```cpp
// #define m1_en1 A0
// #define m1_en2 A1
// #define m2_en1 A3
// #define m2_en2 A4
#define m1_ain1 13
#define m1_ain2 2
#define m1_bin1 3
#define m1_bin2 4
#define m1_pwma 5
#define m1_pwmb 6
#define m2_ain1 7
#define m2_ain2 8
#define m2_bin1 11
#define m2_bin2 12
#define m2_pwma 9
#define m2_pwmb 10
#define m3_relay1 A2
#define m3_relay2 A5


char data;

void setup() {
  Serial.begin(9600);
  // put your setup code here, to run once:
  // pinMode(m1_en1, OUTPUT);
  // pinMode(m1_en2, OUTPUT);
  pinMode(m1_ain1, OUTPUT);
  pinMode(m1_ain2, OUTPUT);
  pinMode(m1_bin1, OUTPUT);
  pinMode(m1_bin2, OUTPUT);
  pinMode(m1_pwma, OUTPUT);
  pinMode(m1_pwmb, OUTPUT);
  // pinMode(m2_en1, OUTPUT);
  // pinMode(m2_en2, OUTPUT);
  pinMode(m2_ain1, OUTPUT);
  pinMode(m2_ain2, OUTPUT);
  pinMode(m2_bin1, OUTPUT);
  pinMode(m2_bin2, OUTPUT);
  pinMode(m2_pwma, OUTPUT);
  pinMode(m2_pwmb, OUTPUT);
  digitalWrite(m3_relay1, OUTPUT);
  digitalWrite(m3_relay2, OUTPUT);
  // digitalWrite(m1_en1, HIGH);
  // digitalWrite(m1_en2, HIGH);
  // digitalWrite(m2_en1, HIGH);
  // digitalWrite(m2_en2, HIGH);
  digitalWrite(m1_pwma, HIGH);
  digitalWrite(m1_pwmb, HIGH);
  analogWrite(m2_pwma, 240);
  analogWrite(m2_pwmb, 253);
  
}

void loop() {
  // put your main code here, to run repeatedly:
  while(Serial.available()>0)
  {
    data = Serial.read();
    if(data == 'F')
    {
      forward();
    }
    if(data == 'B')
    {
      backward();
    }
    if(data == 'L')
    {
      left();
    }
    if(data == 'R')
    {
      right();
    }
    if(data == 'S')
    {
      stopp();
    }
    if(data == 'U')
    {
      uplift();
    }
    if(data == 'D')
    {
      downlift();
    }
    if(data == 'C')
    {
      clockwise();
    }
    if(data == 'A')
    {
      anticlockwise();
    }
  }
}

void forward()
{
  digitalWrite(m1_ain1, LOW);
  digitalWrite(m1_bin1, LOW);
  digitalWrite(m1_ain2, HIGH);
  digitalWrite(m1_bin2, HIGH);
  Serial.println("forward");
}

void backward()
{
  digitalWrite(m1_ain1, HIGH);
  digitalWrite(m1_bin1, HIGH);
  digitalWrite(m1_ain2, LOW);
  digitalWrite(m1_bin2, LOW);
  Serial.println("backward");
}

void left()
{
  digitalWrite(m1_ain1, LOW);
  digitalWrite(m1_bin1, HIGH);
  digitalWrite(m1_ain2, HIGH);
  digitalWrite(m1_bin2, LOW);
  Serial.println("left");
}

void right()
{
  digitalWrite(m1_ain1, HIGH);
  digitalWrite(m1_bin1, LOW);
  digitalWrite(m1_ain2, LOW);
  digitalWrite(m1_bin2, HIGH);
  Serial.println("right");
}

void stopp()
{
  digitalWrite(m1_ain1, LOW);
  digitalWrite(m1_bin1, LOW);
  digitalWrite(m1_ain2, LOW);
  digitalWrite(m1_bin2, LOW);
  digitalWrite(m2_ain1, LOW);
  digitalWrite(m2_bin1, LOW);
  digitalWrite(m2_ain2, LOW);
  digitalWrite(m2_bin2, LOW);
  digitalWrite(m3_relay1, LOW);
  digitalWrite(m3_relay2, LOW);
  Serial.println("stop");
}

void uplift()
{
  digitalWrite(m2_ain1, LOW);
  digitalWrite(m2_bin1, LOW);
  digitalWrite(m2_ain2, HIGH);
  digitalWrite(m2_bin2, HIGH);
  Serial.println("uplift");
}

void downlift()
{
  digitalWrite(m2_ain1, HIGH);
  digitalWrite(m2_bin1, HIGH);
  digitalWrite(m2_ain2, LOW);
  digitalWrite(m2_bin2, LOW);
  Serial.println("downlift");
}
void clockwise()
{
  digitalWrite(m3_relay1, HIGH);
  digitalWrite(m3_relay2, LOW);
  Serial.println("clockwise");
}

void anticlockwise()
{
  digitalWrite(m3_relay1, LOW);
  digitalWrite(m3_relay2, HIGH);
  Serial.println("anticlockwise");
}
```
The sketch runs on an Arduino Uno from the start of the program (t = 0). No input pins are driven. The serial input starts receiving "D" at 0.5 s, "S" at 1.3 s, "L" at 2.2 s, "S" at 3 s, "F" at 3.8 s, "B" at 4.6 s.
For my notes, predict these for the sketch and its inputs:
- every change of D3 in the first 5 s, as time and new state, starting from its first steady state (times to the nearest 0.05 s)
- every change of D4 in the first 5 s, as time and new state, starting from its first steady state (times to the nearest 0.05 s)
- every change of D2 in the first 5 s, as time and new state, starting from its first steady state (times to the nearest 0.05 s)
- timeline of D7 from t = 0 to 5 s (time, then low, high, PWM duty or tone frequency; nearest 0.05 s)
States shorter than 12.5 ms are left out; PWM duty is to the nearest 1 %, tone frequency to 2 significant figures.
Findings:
0 s low; 2.2 s high; 3 s low; 4.6 s high
0 s low; 3.8 s high; 4.6 s low
0 s low; 2.2 s high; 3 s low; 3.8 s high; 4.6 s low
0 s low; 0.5 s high; 1.3 s low
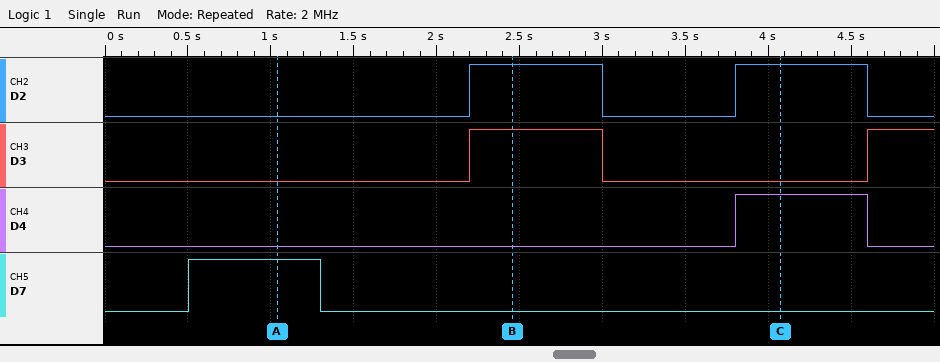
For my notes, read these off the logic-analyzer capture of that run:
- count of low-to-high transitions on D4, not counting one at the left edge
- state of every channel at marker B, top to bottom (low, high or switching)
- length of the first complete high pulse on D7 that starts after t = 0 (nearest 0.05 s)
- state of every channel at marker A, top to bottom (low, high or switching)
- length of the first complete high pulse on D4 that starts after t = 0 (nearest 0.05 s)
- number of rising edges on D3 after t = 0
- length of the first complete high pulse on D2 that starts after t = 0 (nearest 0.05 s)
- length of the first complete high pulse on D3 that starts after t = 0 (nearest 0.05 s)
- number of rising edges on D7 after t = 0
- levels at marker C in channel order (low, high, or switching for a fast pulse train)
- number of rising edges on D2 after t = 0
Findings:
1
D2 high, D3 high, D4 low, D7 low
0.80 s
D2 low, D3 low, D4 low, D7 high
0.80 s
2
0.80 s
0.80 s
1
D2 high, D3 low, D4 high, D7 low
2
